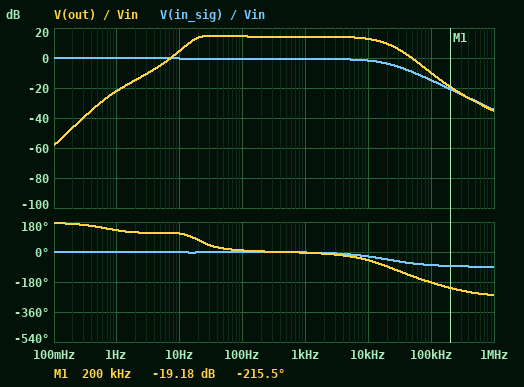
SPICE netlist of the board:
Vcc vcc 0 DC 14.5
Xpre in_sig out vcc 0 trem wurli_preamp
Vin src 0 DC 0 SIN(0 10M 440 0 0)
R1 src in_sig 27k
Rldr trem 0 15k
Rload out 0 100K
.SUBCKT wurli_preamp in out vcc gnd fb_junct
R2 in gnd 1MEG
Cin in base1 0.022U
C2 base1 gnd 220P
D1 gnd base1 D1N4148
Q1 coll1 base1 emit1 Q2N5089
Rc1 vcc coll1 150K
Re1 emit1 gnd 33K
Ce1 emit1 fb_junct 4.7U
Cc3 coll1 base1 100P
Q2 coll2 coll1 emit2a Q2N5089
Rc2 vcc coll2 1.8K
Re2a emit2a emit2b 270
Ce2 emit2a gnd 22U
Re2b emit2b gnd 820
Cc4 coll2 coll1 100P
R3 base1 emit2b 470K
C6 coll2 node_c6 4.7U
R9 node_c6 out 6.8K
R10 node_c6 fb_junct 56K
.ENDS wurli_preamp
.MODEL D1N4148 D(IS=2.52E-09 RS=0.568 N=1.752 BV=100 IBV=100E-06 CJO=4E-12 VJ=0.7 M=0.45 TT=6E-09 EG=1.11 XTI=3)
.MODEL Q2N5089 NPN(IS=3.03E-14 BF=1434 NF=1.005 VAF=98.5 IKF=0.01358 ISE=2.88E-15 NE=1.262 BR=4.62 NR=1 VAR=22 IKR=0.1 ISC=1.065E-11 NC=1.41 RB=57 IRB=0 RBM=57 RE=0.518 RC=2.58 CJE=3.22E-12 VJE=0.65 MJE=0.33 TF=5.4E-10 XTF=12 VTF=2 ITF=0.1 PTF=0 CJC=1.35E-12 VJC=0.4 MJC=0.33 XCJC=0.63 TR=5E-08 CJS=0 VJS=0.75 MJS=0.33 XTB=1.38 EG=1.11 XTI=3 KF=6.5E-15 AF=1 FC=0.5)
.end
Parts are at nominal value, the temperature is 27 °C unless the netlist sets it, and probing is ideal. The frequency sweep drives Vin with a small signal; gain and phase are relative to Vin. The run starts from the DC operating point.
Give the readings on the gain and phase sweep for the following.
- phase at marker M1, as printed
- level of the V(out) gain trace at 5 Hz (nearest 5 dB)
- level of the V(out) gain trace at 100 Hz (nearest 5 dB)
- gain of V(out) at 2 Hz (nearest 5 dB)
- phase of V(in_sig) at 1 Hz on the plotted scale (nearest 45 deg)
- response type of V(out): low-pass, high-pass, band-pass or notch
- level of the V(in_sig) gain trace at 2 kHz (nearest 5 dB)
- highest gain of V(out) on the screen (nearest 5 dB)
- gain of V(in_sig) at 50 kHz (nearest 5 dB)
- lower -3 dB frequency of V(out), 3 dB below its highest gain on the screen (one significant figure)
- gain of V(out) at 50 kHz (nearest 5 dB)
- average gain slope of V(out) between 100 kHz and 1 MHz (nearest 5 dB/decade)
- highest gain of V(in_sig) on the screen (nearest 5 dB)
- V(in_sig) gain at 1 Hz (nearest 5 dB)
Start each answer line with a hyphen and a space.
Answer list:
- -215.5 deg
- -5 dB
- 15 dB
- -15 dB
- 0 deg
- band-pass
- 0 dB
- 15 dB
- -10 dB
- 20 Hz
- 0 dB
- -25 dB/decade
- 0 dB
- 0 dB
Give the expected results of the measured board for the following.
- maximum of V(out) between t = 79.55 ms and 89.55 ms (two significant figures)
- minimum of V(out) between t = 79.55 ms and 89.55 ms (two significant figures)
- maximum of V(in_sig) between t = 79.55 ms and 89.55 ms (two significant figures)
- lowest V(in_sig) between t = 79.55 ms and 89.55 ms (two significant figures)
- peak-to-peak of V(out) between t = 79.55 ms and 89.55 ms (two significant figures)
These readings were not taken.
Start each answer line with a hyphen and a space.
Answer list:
- 52 mV
- -52 mV
- 9.2 mV
- -9.2 mV
- 100 mV
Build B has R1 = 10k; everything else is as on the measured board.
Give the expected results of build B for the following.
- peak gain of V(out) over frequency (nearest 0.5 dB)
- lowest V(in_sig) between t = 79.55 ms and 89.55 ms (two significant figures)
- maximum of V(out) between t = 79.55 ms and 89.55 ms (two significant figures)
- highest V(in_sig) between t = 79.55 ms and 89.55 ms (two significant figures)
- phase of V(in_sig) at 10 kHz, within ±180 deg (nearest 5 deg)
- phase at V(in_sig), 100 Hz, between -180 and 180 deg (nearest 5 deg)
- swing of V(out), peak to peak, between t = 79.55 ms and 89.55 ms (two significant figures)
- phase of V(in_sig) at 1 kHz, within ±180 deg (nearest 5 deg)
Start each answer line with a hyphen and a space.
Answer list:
- 15.5 dB
- -9.7 mV
- 54 mV
- 9.7 mV
- -10 deg
- 0 deg
- 110 mV
- 0 deg
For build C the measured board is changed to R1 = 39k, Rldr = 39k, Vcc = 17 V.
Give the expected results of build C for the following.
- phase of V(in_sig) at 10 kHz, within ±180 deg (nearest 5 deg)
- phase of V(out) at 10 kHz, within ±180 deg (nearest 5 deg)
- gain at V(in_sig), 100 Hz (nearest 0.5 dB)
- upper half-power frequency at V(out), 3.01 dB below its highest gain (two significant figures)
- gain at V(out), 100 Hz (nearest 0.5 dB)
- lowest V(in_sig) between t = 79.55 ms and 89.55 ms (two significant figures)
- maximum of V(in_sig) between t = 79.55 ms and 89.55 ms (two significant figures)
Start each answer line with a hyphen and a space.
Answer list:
- -35 deg
- -60 deg
- -1.0 dB
- 12 kHz
- 10.0 dB
- -8.9 mV
- 8.9 mV
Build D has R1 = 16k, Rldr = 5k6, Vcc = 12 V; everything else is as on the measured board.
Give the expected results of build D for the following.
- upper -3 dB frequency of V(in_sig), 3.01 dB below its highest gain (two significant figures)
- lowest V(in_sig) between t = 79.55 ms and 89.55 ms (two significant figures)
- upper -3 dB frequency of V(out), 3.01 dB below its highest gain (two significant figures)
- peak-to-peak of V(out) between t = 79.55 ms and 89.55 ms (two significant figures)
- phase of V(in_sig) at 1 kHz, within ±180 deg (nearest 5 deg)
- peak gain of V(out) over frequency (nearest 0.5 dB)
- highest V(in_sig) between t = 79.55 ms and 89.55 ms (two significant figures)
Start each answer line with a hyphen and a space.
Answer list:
- 30 kHz
- -9.5 mV
- 9.7 kHz
- 210 mV
- 0 deg
- 22.5 dB
- 9.5 mV
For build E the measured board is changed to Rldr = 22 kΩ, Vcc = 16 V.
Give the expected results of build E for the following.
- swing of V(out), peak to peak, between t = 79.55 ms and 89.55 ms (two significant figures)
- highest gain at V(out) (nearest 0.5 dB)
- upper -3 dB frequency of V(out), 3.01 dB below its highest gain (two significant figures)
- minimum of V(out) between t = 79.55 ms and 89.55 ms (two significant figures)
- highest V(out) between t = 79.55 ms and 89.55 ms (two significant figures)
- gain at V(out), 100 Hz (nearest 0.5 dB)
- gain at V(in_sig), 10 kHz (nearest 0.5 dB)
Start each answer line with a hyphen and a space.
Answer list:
- 84 mV
- 13.0 dB
- 14 kHz
- -42 mV
- 42 mV
- 12.5 dB
- -1.5 dB
